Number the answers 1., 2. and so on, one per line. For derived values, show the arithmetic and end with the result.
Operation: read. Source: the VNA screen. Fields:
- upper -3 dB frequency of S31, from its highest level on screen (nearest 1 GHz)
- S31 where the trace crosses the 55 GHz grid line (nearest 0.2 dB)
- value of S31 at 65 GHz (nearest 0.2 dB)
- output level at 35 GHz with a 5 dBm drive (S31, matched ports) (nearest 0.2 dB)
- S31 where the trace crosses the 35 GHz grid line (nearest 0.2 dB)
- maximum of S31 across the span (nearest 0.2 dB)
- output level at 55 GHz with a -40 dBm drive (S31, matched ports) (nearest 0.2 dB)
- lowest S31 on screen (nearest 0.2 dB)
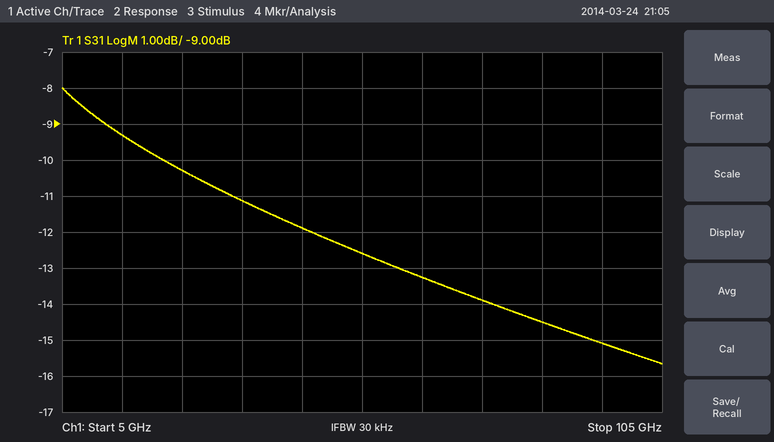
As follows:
1. 33 GHz
2. -12.6 dB
3. -13.2 dB
4. 5 dBm + (-11.2 dB) = -6.2 dBm
5. -11.2 dB
6. -8.0 dB
7. -40 dBm + (-12.6 dB) = -52.6 dBm
8. -15.6 dB
